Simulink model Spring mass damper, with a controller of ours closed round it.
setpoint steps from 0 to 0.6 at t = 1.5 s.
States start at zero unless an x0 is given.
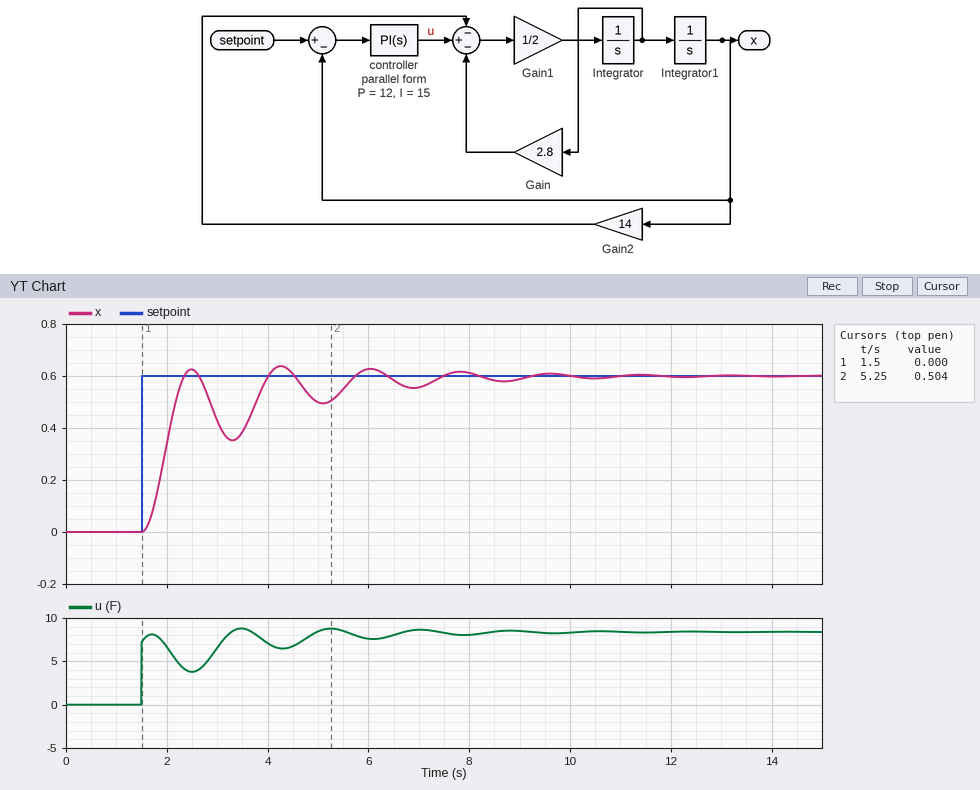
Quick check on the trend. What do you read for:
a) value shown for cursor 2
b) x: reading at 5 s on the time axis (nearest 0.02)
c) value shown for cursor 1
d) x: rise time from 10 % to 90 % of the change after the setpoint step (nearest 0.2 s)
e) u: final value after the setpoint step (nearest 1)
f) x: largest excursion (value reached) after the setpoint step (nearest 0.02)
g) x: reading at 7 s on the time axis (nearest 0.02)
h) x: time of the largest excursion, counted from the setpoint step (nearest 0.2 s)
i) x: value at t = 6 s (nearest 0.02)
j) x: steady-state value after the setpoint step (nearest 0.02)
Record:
0.504
0.50
0.000
0.6 s
8
0.64
0.56
2.8 s
0.62
0.60
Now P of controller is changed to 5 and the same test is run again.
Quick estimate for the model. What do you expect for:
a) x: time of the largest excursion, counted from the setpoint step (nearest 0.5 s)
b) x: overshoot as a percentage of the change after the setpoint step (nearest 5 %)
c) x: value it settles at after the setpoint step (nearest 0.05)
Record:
3.5 s
10 %
0.60
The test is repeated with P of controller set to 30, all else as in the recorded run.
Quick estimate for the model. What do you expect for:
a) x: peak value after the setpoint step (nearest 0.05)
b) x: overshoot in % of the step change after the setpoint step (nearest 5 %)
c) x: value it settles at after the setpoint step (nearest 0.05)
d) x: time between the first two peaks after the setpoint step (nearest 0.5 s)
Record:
0.75
25 %
0.60
1.5 s
